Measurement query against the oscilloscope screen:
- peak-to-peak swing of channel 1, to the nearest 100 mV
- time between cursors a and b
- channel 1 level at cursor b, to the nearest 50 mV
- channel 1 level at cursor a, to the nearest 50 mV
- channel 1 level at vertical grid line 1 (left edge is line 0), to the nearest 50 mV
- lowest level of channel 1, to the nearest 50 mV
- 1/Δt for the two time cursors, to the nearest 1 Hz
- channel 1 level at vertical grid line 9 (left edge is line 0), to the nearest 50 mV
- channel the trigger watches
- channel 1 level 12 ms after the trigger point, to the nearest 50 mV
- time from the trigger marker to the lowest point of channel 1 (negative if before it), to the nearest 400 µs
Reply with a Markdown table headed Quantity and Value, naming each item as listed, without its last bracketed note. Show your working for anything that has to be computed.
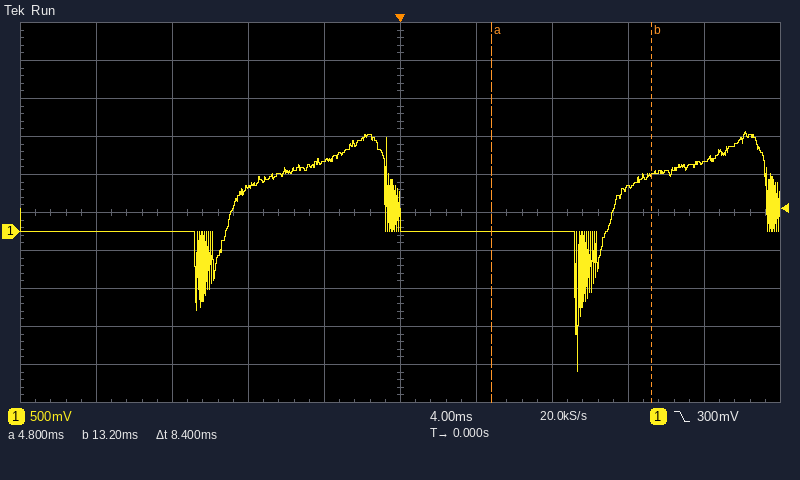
| Quantity | Value |
|---|---|
| peak-to-peak swing of channel 1, to the nearest 100 mV | 3.20 V |
| time between cursors a and b | 8.4 ms |
| channel 1 level at cursor b, to the nearest 50 mV | 750 mV |
| channel 1 level at cursor a, to the nearest 50 mV | 0 mV |
| channel 1 level at vertical grid line 1 (left edge is line 0), to the nearest 50 mV | 0 mV |
| lowest level of channel 1, to the nearest 50 mV | -1.85 V |
| 1/Δt for the two time cursors, to the nearest 1 Hz | 1 / 8.4 ms ≈ 119 Hz |
| channel 1 level at vertical grid line 9 (left edge is line 0), to the nearest 50 mV | 900 mV |
| channel the trigger watches | channel 1 |
| channel 1 level 12 ms after the trigger point, to the nearest 50 mV | 550 mV |
| time from the trigger marker to the lowest point of channel 1 (negative if before it), to the nearest 400 µs | +9.2 ms |
